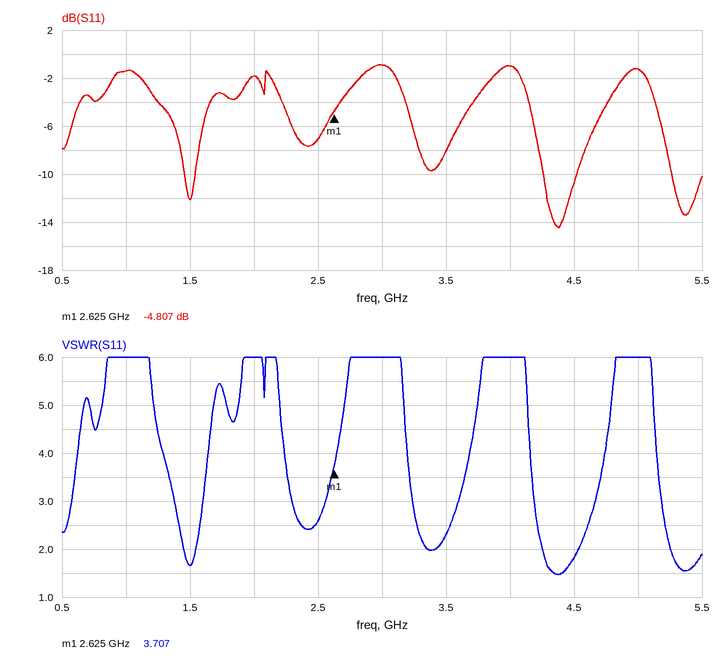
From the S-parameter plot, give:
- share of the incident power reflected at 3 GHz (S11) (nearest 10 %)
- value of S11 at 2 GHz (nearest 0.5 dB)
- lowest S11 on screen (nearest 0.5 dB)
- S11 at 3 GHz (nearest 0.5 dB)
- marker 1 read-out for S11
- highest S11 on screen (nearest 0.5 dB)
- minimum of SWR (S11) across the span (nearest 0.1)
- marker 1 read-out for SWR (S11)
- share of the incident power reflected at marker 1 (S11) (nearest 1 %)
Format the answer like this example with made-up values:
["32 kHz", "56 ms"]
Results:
["80 %", "-2.0 dB", "-14.5 dB", "-1.0 dB", "-4.807 dB", "-1.0 dB", "1.5", "3.707", "33 %"]
